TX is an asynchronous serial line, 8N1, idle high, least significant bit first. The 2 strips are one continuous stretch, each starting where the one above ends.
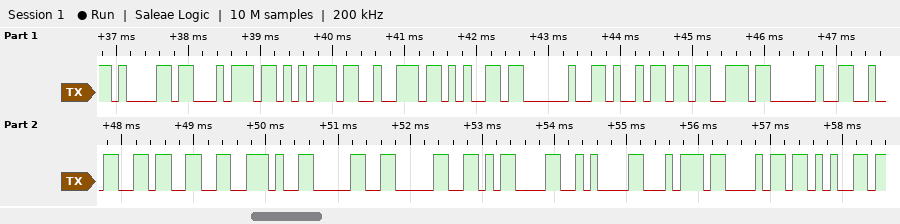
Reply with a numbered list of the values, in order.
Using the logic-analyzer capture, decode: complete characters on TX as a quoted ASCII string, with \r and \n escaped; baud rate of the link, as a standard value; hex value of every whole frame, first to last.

1. "ature is 23.00\r\nthe"
2. 9600 baud
3. 61 74 75 72 65 20 69 73 20 32 33 2E 30 30 0D 0A 74 68 65
